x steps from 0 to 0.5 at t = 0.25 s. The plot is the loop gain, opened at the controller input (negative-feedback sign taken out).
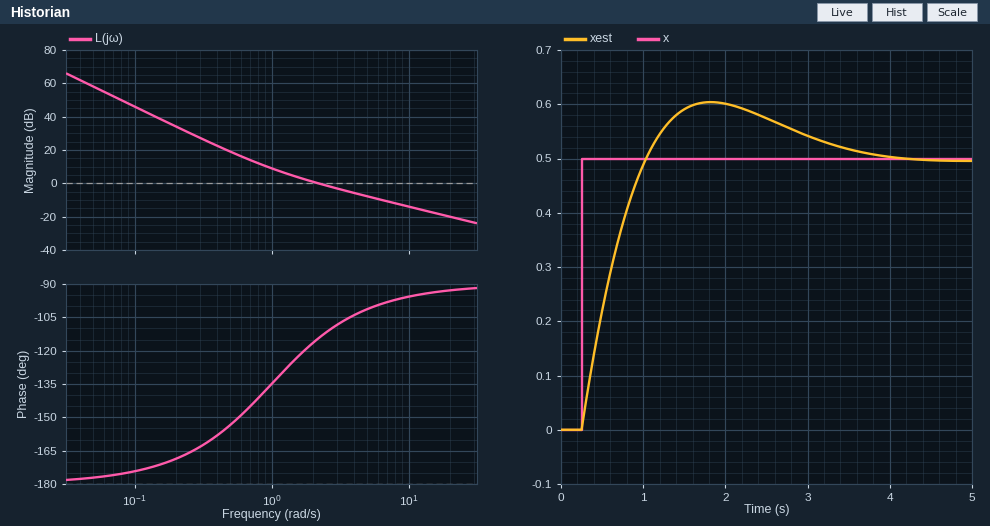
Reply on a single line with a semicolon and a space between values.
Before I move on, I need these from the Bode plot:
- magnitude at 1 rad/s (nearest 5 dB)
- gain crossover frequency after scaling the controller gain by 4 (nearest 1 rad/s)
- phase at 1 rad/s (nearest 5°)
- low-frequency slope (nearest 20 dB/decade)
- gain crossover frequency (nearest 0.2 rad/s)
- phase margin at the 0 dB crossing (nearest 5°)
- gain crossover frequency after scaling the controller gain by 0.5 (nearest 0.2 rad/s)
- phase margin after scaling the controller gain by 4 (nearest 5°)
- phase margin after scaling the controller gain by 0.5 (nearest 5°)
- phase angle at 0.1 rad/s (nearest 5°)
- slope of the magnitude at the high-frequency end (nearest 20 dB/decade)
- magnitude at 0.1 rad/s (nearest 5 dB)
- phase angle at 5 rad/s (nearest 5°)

10 dB; 8 rad/s; -135°; -40 dB/decade; 2.2 rad/s; 65°; 1.2 rad/s; 85°; 50°; -175°; -20 dB/decade; 45 dB; -100°
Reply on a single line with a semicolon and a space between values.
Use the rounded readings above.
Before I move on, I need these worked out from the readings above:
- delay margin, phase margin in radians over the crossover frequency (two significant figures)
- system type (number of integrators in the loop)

0.52 s; 2
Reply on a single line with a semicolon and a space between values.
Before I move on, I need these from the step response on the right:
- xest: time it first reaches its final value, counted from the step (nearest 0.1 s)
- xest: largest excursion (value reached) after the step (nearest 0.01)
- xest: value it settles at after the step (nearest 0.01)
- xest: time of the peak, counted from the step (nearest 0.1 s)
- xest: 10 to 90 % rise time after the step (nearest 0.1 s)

0.8 s; 0.60; 0.50; 1.6 s; 0.6 s
